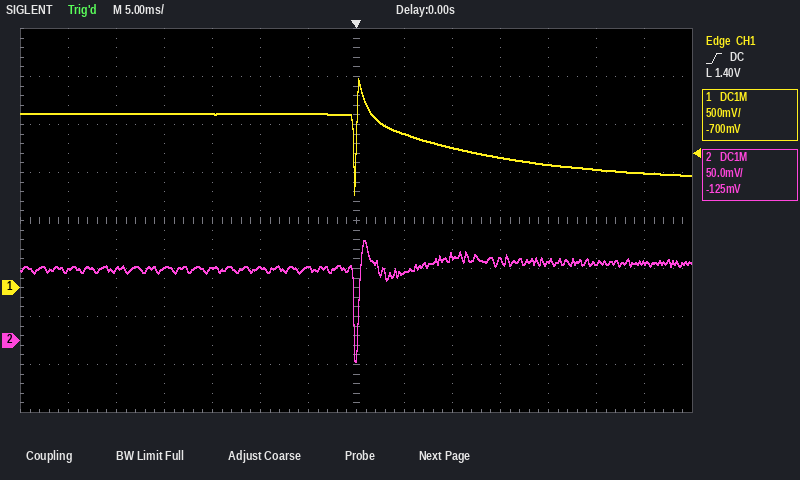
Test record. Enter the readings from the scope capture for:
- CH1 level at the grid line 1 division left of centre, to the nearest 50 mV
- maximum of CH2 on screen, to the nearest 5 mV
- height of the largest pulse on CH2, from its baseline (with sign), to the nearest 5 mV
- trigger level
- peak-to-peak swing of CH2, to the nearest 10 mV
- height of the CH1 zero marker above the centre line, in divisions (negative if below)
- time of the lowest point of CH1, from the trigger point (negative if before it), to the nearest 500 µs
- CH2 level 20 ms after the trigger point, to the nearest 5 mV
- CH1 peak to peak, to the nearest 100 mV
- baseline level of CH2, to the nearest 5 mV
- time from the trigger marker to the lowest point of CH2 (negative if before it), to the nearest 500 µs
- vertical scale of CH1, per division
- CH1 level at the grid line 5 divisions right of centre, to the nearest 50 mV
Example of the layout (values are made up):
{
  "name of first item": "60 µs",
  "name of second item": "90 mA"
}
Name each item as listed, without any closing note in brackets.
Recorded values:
{
  "CH1 level at the grid line 1 division left of centre, to the nearest 50 mV": "1.80 V",
  "maximum of CH2 on screen, to the nearest 5 mV": "105 mV",
  "height of the largest pulse on CH2, from its baseline (with sign), to the nearest 5 mV": "-100 mV",
  "trigger level": "1.40 V",
  "peak-to-peak swing of CH2, to the nearest 10 mV": "130 mV",
  "height of the CH1 zero marker above the centre line, in divisions": "-1.4 div",
  "time of the lowest point of CH1, from the trigger point (negative if before it), to the nearest 500 µs": "0.0 ms",
  "CH2 level 20 ms after the trigger point, to the nearest 5 mV": "80 mV",
  "CH1 peak to peak, to the nearest 100 mV": "1.20 V",
  "baseline level of CH2, to the nearest 5 mV": "75 mV",
  "time from the trigger marker to the lowest point of CH2 (negative if before it), to the nearest 500 µs": "0.0 ms",
  "vertical scale of CH1, per division": "500 mV",
  "CH1 level at the grid line 5 divisions right of centre, to the nearest 50 mV": "1.25 V"
}
